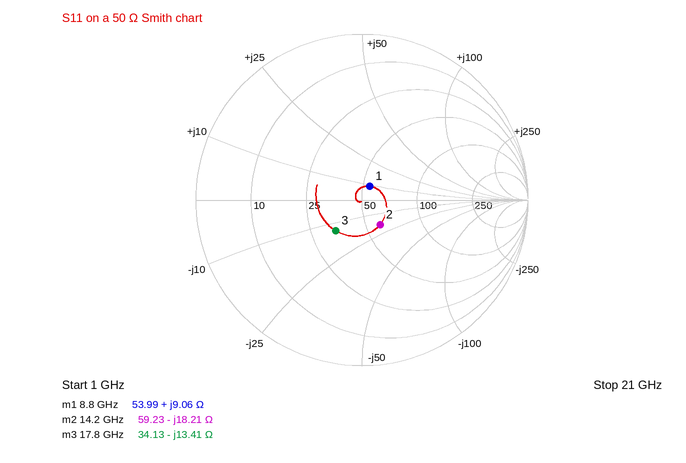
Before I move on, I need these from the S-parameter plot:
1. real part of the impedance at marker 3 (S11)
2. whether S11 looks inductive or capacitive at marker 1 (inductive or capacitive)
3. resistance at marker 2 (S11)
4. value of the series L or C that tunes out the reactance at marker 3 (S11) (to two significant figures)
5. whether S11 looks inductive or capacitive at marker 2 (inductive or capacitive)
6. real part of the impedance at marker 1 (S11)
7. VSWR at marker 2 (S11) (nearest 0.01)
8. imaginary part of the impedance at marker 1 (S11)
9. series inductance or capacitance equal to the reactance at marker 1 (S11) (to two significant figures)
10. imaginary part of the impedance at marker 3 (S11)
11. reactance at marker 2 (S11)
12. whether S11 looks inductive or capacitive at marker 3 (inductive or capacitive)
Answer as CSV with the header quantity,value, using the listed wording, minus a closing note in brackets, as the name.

quantity,value
real part of the impedance at marker 3,34.13 Ω
whether S11 looks inductive or capacitive at marker 1,inductive
resistance at marker 2,59.23 Ω
value of the series L or C that tunes out the reactance at marker 3 (S11),120 pH
whether S11 looks inductive or capacitive at marker 2,capacitive
real part of the impedance at marker 1,53.99 Ω
VSWR at marker 2 (S11),1.45
imaginary part of the impedance at marker 1,+9.06 Ω
series inductance or capacitance equal to the reactance at marker 1 (S11),160 pH
imaginary part of the impedance at marker 3,-13.41 Ω
reactance at marker 2,-18.21 Ω
whether S11 looks inductive or capacitive at marker 3,capacitive
